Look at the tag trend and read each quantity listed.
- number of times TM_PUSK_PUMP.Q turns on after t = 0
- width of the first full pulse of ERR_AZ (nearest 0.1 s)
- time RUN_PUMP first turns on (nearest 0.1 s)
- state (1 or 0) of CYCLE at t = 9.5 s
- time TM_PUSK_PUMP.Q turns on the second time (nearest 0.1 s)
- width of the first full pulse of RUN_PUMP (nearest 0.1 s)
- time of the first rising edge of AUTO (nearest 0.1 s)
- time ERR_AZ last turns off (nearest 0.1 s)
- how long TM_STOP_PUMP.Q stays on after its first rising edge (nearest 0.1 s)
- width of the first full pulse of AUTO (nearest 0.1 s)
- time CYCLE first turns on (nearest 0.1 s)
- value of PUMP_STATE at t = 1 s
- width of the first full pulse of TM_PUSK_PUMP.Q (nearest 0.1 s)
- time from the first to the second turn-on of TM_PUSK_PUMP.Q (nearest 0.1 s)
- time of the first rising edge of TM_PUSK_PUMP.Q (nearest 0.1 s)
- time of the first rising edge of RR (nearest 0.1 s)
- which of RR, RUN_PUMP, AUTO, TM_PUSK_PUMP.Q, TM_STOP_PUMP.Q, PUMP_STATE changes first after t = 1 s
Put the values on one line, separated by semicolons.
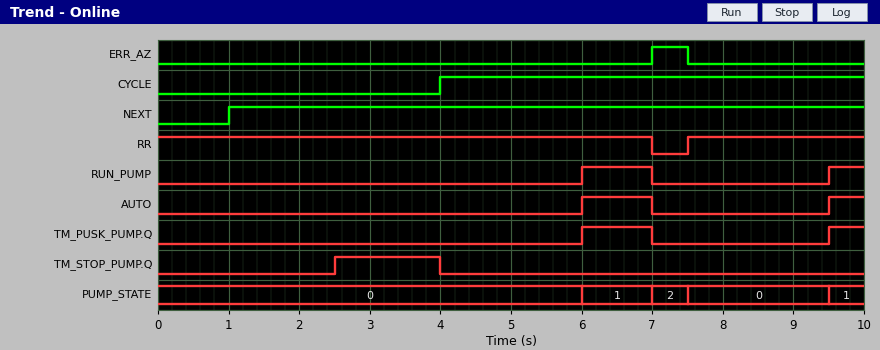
2; 0.5 s; 6.0 s; 1; 9.5 s; 1.0 s; 6.0 s; 7.5 s; 1.5 s; 1.0 s; 4.0 s; 0; 1.0 s; 3.5 s; 6.0 s; 7.5 s; TM_STOP_PUMP.Q
